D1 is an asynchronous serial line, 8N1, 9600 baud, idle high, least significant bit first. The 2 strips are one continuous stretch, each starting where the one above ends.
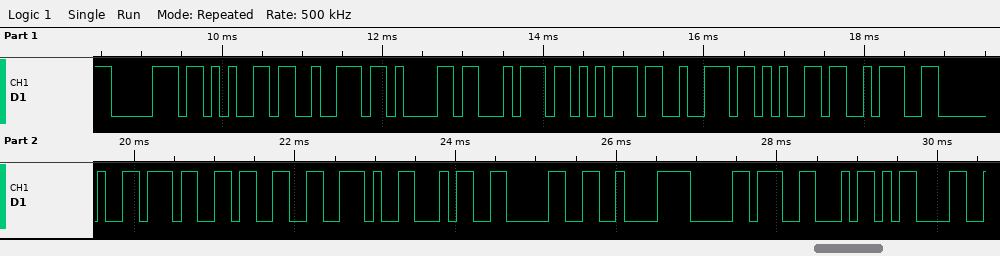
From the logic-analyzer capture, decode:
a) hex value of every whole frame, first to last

70 65 72 61 74 75 72 65 3A 20 37 33 2E 34 30 C2 B0 46 0D
